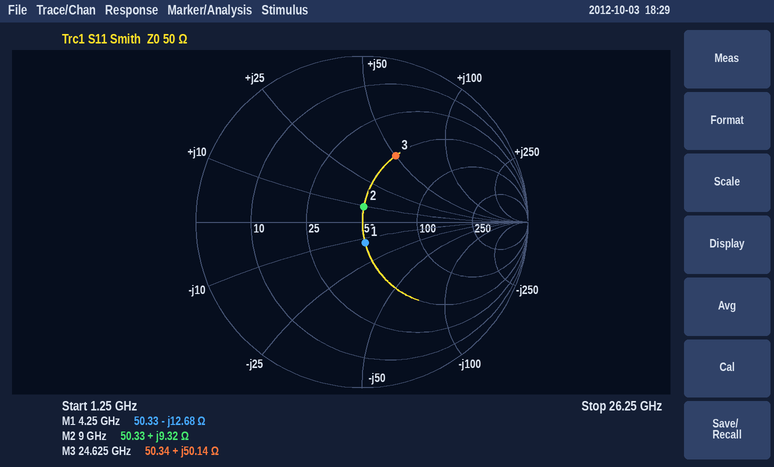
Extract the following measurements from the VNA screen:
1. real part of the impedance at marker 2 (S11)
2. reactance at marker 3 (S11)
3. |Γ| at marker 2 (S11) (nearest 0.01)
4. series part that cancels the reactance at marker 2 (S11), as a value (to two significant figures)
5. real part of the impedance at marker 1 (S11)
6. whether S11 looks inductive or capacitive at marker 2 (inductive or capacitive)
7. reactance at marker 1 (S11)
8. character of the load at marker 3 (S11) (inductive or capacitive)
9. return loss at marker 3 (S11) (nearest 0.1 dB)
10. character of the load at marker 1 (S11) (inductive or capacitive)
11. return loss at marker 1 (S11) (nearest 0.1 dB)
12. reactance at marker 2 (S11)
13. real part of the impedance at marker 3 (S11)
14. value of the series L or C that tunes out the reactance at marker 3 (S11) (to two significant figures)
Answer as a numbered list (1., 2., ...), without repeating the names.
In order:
1. 50.33 Ω
2. +50.14 Ω
3. 0.09
4. 1.9 pF
5. 50.33 Ω
6. inductive
7. -12.68 Ω
8. inductive
9. 7.0 dB
10. capacitive
11. 18.0 dB
12. +9.32 Ω
13. 50.34 Ω
14. 130 fF
